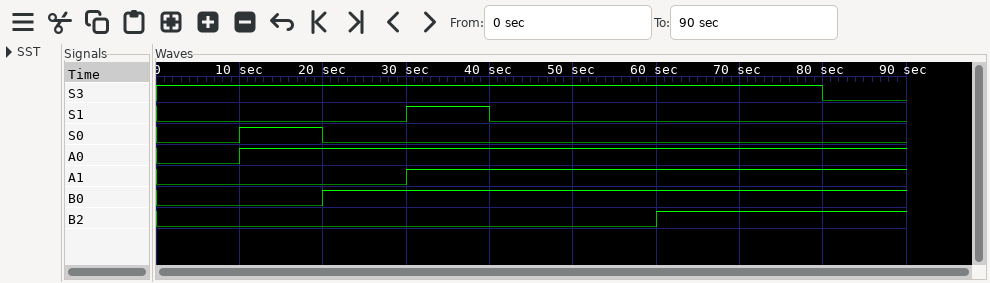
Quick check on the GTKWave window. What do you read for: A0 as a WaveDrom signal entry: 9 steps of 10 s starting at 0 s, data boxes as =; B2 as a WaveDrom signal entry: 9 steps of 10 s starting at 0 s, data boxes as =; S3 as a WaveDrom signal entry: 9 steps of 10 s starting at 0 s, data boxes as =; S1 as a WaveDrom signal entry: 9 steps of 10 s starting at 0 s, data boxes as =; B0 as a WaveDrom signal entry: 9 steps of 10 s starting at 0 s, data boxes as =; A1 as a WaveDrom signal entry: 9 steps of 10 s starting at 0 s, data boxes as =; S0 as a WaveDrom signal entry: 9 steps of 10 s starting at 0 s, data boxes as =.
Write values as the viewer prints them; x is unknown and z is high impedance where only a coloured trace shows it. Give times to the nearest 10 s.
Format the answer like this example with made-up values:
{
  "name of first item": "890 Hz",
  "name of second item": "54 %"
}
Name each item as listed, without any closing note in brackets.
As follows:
{
  "A0 as a WaveDrom signal entry: 9 steps of 10 s starting at 0 s, data boxes as =": "{name: 'A0', wave: '01.......'}",
  "B2 as a WaveDrom signal entry: 9 steps of 10 s starting at 0 s, data boxes as =": "{name: 'B2', wave: '0.....1..'}",
  "S3 as a WaveDrom signal entry: 9 steps of 10 s starting at 0 s, data boxes as =": "{name: 'S3', wave: '1.......0'}",
  "S1 as a WaveDrom signal entry: 9 steps of 10 s starting at 0 s, data boxes as =": "{name: 'S1', wave: '0..10....'}",
  "B0 as a WaveDrom signal entry: 9 steps of 10 s starting at 0 s, data boxes as =": "{name: 'B0', wave: '0.1......'}",
  "A1 as a WaveDrom signal entry: 9 steps of 10 s starting at 0 s, data boxes as =": "{name: 'A1', wave: '0..1.....'}",
  "S0 as a WaveDrom signal entry: 9 steps of 10 s starting at 0 s, data boxes as =": "{name: 'S0', wave: '010......'}"
}
